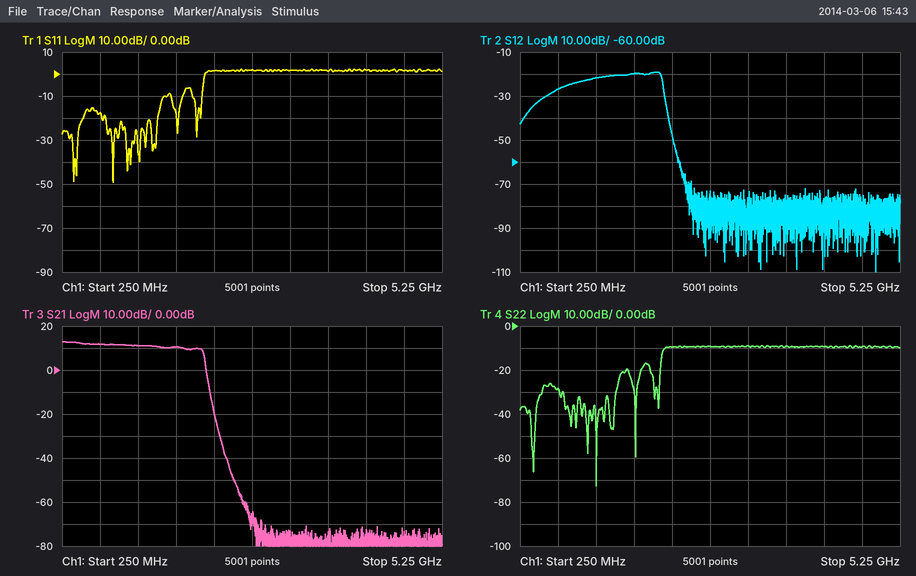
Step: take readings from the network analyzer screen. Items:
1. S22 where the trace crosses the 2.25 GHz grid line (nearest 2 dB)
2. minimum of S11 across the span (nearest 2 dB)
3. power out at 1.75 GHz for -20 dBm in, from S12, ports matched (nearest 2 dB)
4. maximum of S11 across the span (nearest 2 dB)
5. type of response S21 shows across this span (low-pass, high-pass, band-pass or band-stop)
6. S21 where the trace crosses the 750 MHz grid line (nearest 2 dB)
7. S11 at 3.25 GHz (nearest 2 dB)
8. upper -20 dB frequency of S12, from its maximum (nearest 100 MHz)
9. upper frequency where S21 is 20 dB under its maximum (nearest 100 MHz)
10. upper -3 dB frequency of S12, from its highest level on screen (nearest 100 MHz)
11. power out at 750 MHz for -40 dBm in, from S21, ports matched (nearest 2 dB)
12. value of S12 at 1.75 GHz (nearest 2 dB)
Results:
-10 dB
-50 dB
-40 dBm
2 dB
low-pass
12 dB
2 dB
2.2 GHz
2.2 GHz
2.1 GHz
-28 dBm
-20 dB
